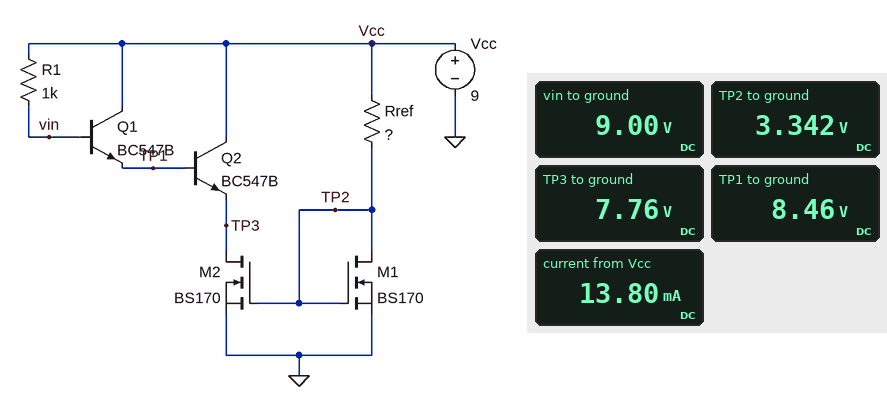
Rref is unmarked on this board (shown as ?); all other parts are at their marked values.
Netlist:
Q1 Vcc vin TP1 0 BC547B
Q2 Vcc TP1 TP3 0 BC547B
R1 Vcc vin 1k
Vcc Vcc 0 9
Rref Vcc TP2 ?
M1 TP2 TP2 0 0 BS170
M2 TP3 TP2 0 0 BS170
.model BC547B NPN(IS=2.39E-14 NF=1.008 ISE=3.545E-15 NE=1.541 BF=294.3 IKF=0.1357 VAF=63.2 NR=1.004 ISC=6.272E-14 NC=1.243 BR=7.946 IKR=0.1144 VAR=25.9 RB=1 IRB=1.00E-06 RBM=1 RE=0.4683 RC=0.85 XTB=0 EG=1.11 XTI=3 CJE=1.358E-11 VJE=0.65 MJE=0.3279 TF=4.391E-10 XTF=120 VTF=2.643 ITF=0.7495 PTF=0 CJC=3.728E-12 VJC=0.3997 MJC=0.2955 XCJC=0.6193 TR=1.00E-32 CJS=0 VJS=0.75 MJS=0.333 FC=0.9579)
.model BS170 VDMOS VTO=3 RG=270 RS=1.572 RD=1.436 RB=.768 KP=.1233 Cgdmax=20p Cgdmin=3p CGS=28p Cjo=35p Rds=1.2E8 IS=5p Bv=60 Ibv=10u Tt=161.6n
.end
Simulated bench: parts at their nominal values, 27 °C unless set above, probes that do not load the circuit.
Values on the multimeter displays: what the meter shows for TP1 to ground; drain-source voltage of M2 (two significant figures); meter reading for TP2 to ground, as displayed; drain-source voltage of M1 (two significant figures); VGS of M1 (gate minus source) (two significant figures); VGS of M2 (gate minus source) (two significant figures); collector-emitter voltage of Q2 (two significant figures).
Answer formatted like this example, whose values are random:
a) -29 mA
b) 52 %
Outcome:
a) 8.46 V
b) 7.8 V
c) 3.342 V
d) 3.3 V
e) 3.3 V
f) 3.3 V
g) 1.2 V
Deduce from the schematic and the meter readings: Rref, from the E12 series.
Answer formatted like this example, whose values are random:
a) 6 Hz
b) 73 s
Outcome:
a) 820 Ω
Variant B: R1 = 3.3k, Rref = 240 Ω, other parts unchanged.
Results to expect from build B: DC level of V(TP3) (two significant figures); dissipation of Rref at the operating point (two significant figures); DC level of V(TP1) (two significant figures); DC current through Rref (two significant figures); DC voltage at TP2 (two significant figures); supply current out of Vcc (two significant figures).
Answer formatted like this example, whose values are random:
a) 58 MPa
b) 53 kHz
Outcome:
a) 7.7 V
b) 120 mW
c) 8.4 V
d) 22 mA
e) 3.6 V
f) 45 mA
